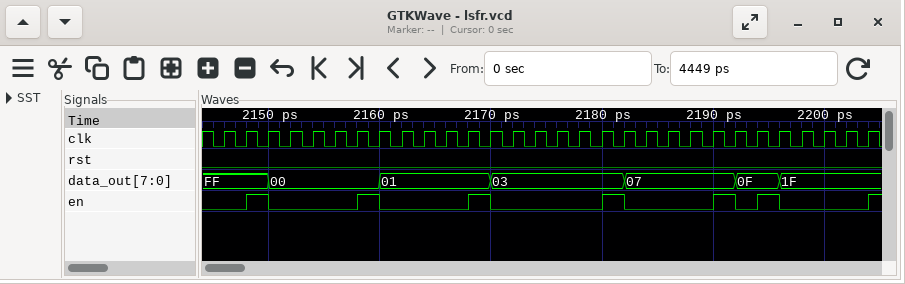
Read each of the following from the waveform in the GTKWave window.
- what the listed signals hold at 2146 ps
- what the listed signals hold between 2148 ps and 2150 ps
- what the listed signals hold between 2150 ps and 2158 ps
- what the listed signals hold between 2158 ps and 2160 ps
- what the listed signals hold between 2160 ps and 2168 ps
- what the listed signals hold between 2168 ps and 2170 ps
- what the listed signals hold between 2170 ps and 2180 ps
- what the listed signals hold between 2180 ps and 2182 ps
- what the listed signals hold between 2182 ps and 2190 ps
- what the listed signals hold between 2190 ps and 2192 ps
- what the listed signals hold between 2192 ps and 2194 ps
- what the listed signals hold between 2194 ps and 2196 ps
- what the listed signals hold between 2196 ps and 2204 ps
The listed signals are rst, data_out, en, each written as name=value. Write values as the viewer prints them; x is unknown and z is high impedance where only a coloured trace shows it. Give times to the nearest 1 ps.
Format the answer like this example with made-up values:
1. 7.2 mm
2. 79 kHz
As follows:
1. rst=0, data_out=FF, en=0
2. rst=0, data_out=FF, en=1
3. rst=0, data_out=00, en=0
4. rst=0, data_out=00, en=1
5. rst=0, data_out=01, en=0
6. rst=0, data_out=01, en=1
7. rst=0, data_out=03, en=0
8. rst=0, data_out=03, en=1
9. rst=0, data_out=07, en=0
10. rst=0, data_out=07, en=1
11. rst=0, data_out=0F, en=0
12. rst=0, data_out=0F, en=1
13. rst=0, data_out=1F, en=0
